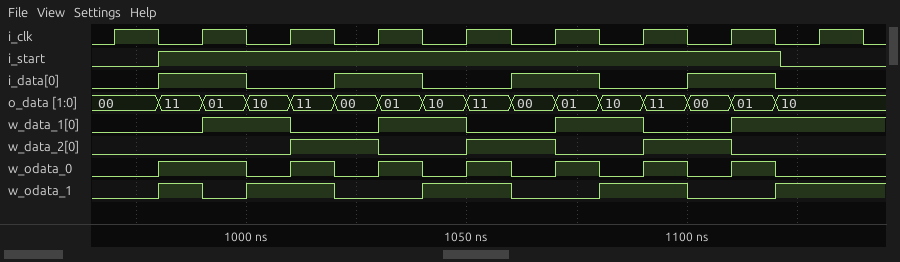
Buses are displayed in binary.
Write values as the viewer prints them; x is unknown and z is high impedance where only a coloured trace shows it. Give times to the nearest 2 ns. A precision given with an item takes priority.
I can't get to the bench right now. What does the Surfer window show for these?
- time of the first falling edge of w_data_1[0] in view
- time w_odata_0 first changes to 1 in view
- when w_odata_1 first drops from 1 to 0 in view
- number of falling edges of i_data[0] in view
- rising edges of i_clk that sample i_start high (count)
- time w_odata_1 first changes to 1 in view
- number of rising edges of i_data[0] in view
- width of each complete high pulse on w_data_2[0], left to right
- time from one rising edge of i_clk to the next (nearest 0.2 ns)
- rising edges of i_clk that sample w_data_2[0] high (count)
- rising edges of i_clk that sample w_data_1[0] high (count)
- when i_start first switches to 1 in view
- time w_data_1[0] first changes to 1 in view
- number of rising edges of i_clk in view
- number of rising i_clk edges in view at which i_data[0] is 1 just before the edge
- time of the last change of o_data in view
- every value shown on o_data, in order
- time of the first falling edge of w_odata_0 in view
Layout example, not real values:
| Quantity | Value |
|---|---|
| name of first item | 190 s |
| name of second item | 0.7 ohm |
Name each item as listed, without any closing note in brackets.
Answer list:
| Quantity | Value |
|---|---|
| time of the first falling edge of w_data_1[0] in view | 1010 ns |
| time w_odata_0 first changes to 1 in view | 980 ns |
| when w_odata_1 first drops from 1 to 0 in view | 990 ns |
| number of falling edges of i_data[0] in view | 4 |
| rising edges of i_clk that sample i_start high | 7 |
| time w_odata_1 first changes to 1 in view | 980 ns |
| number of rising edges of i_data[0] in view | 4 |
| width of each complete high pulse on w_data_2[0], left to right | 20 ns, 20 ns, 20 ns |
| time from one rising edge of i_clk to the next | 20 ns |
| rising edges of i_clk that sample w_data_2[0] high | 3 |
| rising edges of i_clk that sample w_data_1[0] high | 4 |
| when i_start first switches to 1 in view | 980 ns |
| time w_data_1[0] first changes to 1 in view | 990 ns |
| number of rising edges of i_clk in view | 9 |
| number of rising i_clk edges in view at which i_data[0] is 1 just before the edge | 4 |
| time of the last change of o_data in view | 1120 ns |
| every value shown on o_data, in order | 00, 11, 01, 10, 11, 00, 01, 10, 11, 00, 01, 10, 11, 00, 01, 10 |
| time of the first falling edge of w_odata_0 in view | 1000 ns |
